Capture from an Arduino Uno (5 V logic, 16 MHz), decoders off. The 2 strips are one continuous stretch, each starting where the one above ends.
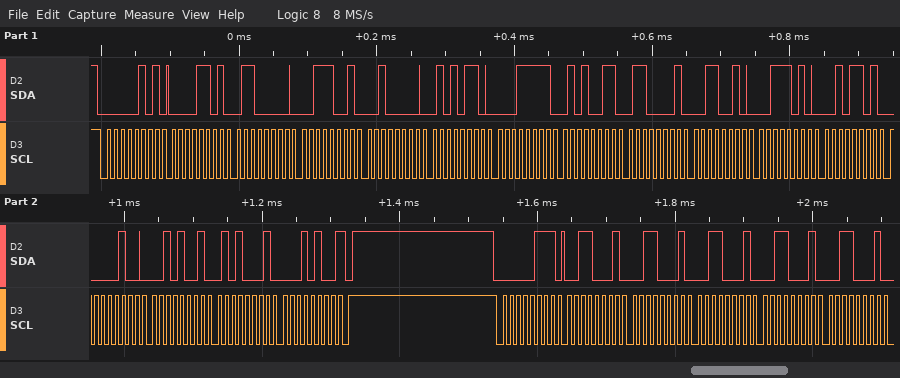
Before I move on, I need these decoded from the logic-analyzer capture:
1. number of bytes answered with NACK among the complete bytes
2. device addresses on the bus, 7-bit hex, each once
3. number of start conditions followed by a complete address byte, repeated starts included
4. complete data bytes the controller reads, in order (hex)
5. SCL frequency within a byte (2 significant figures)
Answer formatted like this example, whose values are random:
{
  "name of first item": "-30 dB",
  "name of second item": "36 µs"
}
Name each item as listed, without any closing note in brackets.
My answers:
{
  "number of bytes answered with NACK among the complete bytes": "1",
  "device addresses on the bus, 7-bit hex, each once": "0x02 0x03",
  "number of start conditions followed by a complete address byte, repeated starts included": "2",
  "complete data bytes the controller reads, in order": "0D 60 39 20 56 1F 53 61 32 3A 2D 04 29 51 14 31 31 31 31 31",
  "SCL frequency within a byte": "100 kHz"
}
